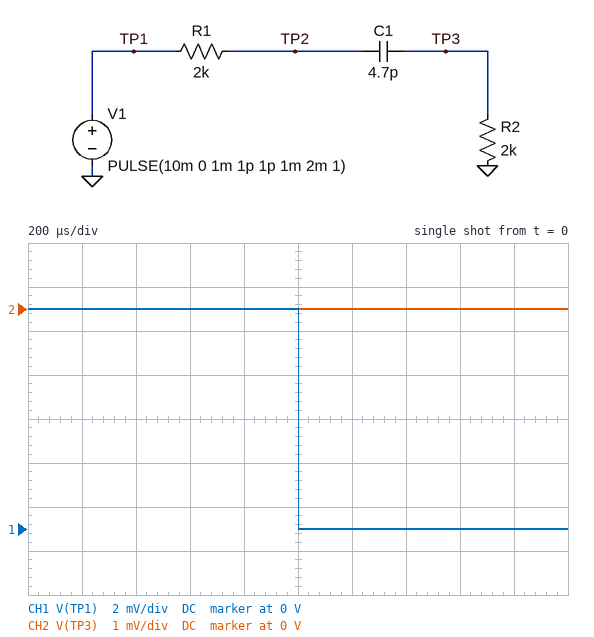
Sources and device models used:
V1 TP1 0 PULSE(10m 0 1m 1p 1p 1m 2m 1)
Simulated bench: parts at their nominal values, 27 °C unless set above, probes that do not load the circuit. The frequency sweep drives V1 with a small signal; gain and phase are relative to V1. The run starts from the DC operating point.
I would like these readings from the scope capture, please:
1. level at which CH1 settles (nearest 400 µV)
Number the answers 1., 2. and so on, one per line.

1. 0 V
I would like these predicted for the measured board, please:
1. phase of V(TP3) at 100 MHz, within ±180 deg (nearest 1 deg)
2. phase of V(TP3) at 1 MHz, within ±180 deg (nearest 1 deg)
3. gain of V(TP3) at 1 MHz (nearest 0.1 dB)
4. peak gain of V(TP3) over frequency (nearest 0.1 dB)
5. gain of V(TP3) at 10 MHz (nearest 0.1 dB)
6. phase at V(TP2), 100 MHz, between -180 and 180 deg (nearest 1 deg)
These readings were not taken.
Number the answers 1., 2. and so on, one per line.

1. 5 deg
2. 83 deg
3. -24.6 dB
4. -6.0 dB
5. -8.4 dB
6. -5 deg
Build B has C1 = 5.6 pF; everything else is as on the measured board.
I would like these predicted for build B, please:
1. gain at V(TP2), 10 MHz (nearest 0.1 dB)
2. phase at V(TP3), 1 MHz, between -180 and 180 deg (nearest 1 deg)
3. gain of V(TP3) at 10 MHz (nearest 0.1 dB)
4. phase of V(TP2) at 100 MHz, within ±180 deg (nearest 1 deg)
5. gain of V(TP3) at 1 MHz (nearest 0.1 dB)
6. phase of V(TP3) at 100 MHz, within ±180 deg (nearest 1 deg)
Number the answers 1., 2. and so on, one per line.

1. -3.0 dB
2. 82 deg
3. -7.8 dB
4. -4 deg
5. -23.1 dB
6. 4 deg
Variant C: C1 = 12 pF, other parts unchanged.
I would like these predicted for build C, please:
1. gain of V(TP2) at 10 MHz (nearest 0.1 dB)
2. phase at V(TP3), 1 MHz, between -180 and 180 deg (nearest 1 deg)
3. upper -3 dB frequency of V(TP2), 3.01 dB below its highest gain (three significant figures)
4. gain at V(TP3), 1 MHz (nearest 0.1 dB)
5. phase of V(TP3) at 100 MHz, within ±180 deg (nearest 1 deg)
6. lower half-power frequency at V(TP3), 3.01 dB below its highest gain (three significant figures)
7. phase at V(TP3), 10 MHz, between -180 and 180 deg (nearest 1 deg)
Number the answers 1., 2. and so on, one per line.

1. -4.9 dB
2. 73 deg
3. 4.69 MHz
4. -16.8 dB
5. 2 deg
6. 3.32 MHz
7. 18 deg
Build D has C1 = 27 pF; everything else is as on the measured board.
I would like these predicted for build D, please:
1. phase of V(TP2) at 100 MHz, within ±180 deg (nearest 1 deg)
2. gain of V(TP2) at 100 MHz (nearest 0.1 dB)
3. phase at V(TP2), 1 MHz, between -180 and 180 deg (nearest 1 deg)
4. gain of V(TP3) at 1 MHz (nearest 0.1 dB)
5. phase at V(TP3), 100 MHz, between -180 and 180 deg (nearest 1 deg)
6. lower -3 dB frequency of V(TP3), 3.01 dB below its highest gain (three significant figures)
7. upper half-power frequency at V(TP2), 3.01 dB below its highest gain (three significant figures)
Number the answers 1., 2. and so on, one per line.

1. -1 deg
2. -6.0 dB
3. -15 deg
4. -11.0 dB
5. 1 deg
6. 1.47 MHz
7. 2.08 MHz
